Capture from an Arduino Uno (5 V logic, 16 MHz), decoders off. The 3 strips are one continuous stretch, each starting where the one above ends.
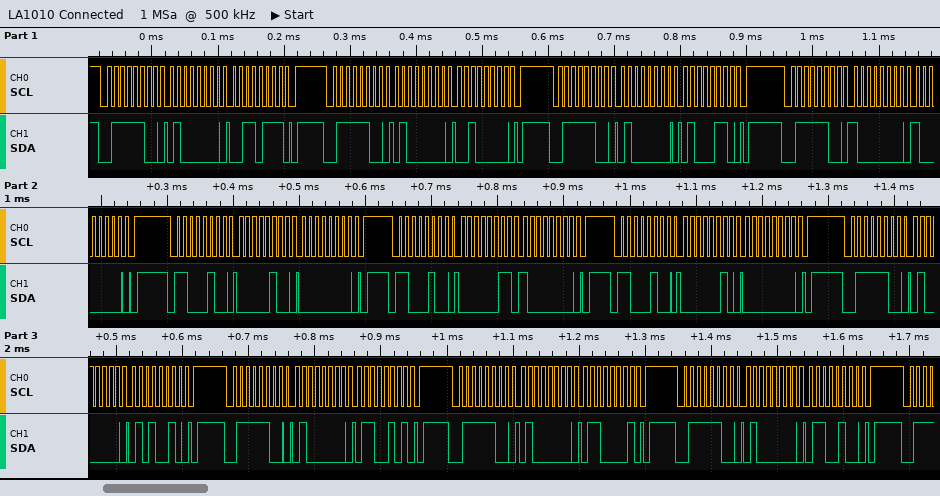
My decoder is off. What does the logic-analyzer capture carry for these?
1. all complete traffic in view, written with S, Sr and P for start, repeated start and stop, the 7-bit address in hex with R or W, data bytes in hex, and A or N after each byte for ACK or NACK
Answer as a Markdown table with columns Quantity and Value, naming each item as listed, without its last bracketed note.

| Quantity | Value |
|---|---|
| all complete traffic in view, written with S, Sr and P for start, repeated start and stop, the 7-bit address in hex with R or W, data bytes in hex, and A or N after each byte for ACK or NACK | S 3EW A 40 A 37 A P S 3EW A 40 A 20 A P S 3EW A 40 A 46 A P S 3EW A 80 A 80 A P S 62W A 04 A 00 A P S 62W A 03 A 80 A P S 62W A 02 A 00 A P S 3EW A 40 A 52 A P S 3EW A 40 A 65 A P S 3EW A 40 A 61 A P S 3EW A 40 A 64 A P |
